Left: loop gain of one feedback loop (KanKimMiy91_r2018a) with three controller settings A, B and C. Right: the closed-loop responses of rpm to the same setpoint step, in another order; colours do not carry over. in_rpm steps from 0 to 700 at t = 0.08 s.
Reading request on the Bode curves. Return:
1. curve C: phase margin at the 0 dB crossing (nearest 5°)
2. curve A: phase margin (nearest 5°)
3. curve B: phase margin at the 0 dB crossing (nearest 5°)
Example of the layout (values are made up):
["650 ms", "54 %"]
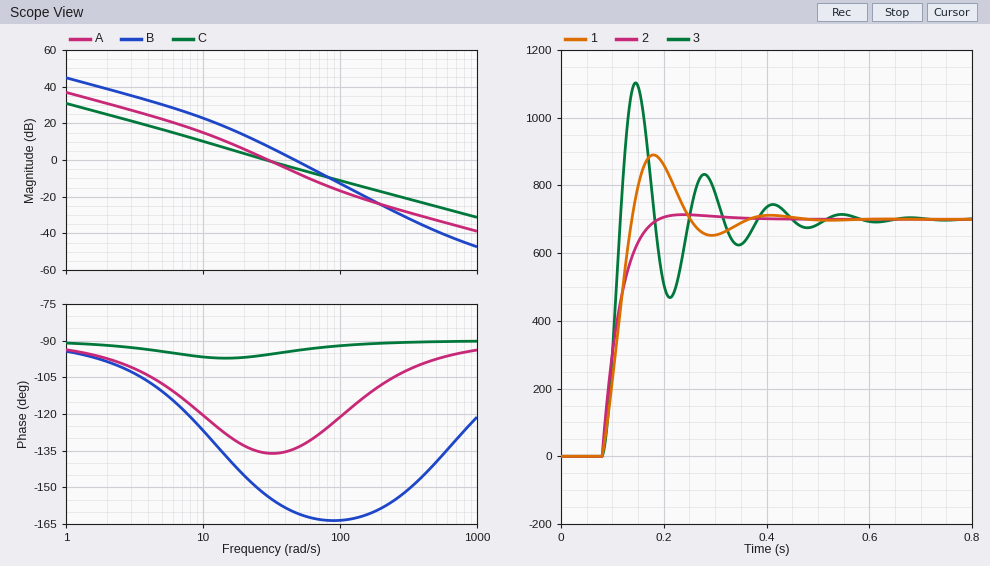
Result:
["85°", "45°", "20°"]
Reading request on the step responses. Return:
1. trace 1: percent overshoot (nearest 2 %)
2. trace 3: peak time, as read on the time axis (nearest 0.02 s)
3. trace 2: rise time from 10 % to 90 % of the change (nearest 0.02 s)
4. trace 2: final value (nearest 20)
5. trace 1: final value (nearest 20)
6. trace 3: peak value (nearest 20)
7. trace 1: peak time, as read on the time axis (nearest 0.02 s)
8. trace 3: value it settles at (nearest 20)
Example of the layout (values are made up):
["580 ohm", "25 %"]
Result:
["28 %", "0.14 s", "0.06 s", "700", "700", "1100", "0.18 s", "700"]
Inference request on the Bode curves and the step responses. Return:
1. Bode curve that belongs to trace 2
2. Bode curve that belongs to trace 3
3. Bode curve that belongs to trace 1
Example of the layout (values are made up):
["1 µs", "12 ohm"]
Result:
["C", "B", "A"]
